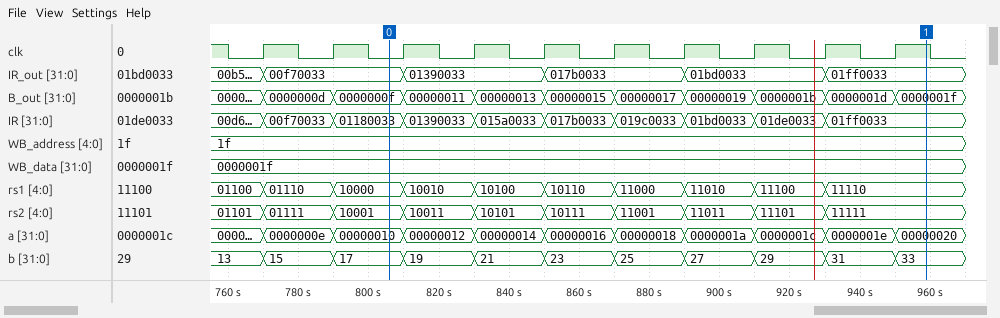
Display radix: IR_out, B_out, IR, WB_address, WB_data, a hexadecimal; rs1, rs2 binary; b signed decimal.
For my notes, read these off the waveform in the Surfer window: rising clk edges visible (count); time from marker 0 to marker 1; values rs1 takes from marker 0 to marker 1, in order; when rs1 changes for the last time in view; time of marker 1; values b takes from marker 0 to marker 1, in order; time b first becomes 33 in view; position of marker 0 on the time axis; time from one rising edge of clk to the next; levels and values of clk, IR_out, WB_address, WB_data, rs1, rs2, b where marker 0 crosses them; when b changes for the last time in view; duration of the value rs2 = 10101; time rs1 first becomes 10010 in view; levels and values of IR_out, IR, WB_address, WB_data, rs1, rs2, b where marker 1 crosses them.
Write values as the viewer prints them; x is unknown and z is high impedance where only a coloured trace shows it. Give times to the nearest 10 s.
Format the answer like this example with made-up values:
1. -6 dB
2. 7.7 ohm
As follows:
1. 10
2. 150 s
3. 10000, 10010, 10100, 10110, 11000, 11010, 11100, 11110
4. 930 s
5. 960 s
6. 17, 19, 21, 23, 25, 27, 29, 31, 33
7. 950 s
8. 810 s
9. 20 s
10. clk=0, IR_out=00f70033, WB_address=1f, WB_data=0000001f, rs1=10000, rs2=10001, b=17
11. 950 s
12. 20 s
13. 810 s
14. IR_out=01ff0033, IR=01ff0033, WB_address=1f, WB_data=0000001f, rs1=11110, rs2=11111, b=33
